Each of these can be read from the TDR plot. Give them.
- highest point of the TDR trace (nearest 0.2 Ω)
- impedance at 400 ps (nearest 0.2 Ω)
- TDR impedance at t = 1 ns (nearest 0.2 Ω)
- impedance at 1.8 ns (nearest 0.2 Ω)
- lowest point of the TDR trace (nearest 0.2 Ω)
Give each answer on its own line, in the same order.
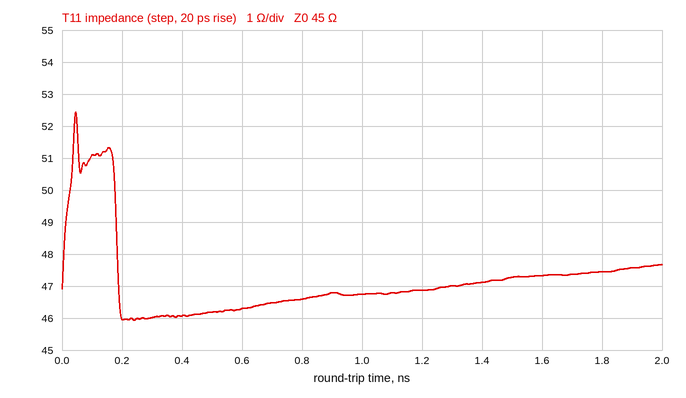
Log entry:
52.4 Ω
46.0 Ω
46.8 Ω
47.4 Ω
46.0 Ω
